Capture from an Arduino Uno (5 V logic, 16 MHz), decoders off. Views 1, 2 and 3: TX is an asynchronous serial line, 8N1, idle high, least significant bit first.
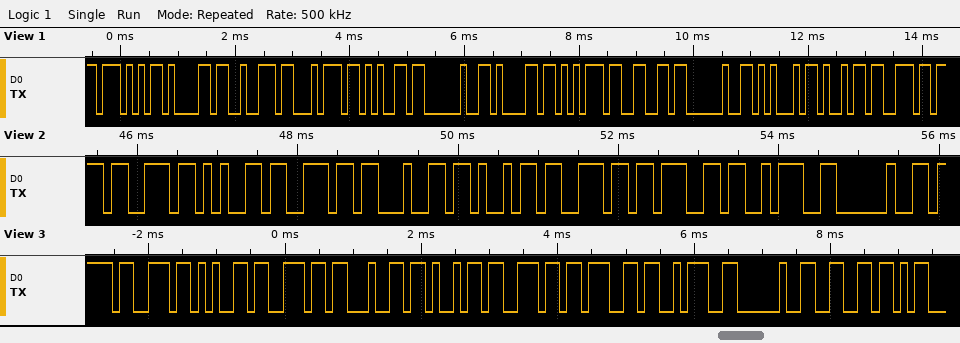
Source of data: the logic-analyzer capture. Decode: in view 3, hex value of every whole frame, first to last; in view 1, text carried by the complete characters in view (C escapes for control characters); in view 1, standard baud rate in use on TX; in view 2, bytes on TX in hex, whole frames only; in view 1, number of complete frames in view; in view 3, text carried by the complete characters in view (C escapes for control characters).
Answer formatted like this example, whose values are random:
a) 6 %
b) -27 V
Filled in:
a) 0x73 0x65 0x6E 0x64 0x69 0x6E 0x67 0x3A 0x20 0x66
b) "Warte auf Ein"
c) 9600 baud
d) 0x73 0x65 0x6E 0x64 0x69 0x6E 0x67 0x3A 0x20
e) 13
f) "sending: f"
